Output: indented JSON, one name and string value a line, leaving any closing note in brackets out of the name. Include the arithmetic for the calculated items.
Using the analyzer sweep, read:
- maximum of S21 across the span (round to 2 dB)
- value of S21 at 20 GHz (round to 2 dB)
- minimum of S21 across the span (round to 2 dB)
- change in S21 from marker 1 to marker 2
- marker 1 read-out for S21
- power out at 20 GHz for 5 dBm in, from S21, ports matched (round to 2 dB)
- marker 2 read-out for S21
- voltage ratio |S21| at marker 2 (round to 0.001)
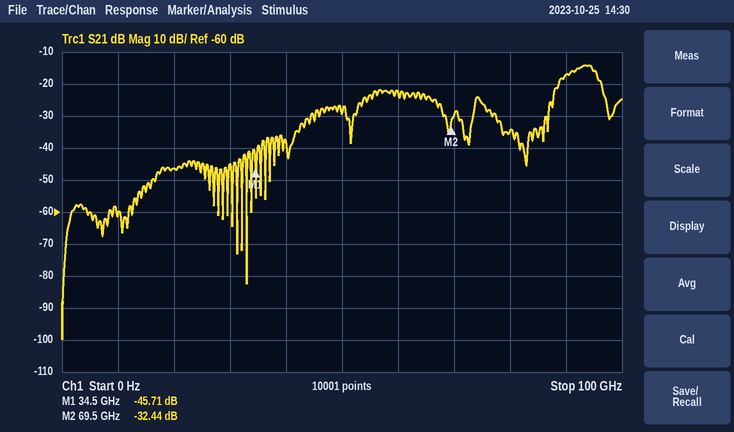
{
  "maximum of S21 across the span": "-14 dB",
  "value of S21 at 20 GHz": "-46 dB",
  "minimum of S21 across the span": "-100 dB",
  "change in S21 from marker 1 to marker 2": "-32.44 − (-45.71) = 13.27 dB",
  "marker 1 read-out for S21": "-45.71 dB",
  "power out at 20 GHz for 5 dBm in, from S21, ports matched": "5 dBm + (-46 dB) = -42 dBm",
  "marker 2 read-out for S21": "-32.44 dB",
  "voltage ratio |S21| at marker 2": "10^(-32.44/20) ≈ 0.024"
}
